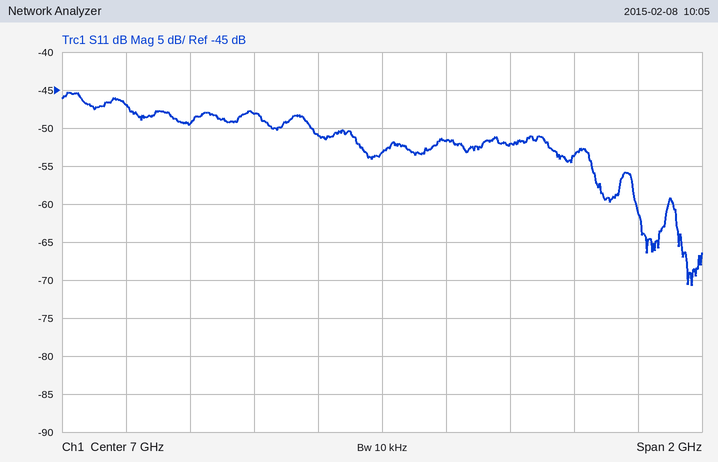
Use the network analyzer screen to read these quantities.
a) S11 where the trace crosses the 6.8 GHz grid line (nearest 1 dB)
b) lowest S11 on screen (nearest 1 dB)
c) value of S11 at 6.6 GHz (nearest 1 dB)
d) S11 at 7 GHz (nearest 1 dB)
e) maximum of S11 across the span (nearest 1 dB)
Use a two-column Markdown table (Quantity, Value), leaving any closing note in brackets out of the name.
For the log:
| Quantity | Value |
|---|---|
| S11 where the trace crosses the 6.8 GHz grid line | -51 dB |
| lowest S11 on screen | -71 dB |
| value of S11 at 6.6 GHz | -48 dB |
| S11 at 7 GHz | -53 dB |
| maximum of S11 across the span | -45 dB |
